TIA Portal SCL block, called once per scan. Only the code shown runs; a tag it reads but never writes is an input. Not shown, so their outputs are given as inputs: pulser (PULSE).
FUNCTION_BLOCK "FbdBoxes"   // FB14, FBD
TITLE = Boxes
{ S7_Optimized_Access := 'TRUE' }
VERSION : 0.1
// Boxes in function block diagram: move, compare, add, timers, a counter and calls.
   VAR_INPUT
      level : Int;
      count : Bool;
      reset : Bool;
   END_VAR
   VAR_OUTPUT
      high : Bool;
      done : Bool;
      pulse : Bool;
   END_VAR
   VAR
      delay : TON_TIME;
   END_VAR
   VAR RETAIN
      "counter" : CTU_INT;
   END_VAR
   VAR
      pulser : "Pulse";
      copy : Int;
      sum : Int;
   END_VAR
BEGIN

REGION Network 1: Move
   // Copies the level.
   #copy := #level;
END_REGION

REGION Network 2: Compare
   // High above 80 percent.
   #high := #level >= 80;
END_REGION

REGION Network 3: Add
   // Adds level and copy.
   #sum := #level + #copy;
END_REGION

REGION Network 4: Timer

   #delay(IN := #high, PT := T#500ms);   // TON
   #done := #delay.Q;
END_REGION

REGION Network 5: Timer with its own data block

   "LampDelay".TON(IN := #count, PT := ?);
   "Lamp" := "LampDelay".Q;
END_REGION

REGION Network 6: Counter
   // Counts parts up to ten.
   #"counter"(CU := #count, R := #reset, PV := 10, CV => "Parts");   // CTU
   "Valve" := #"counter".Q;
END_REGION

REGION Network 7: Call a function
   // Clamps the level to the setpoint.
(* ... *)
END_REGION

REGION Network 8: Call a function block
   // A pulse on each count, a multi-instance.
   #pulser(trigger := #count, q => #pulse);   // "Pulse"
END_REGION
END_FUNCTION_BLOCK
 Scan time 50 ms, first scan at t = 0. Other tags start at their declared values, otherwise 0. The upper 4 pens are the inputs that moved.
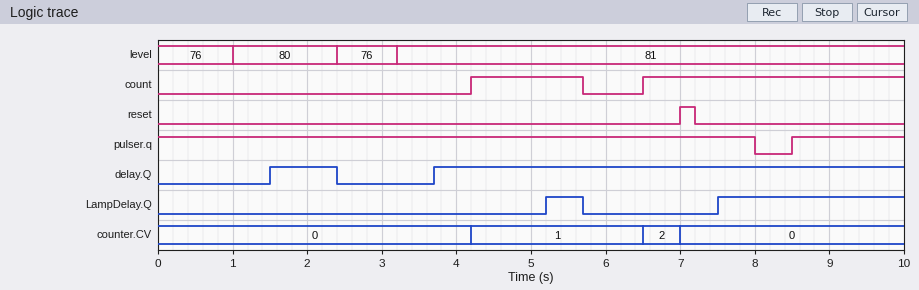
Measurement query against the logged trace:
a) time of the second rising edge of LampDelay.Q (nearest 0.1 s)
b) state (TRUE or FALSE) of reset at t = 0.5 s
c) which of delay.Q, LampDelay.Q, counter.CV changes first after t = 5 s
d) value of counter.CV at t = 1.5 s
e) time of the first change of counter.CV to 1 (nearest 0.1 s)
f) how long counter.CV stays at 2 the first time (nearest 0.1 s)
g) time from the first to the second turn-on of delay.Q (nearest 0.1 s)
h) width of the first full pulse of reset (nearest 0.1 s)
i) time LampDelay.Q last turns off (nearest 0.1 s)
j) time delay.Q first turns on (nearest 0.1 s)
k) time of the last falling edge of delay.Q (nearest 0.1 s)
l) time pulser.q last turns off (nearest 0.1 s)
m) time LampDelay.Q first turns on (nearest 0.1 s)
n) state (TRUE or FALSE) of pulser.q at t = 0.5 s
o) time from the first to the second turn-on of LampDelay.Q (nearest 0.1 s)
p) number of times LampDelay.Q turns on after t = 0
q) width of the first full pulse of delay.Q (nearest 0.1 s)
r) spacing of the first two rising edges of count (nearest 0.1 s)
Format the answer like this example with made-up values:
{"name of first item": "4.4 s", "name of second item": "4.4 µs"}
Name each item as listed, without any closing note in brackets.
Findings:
{"time of the second rising edge of LampDelay.Q": "7.5 s", "state (TRUE or FALSE) of reset at t = 0.5 s": "FALSE", "which of delay.Q, LampDelay.Q, counter.CV changes first after t = 5 s": "LampDelay.Q", "value of counter.CV at t = 1.5 s": "0", "time of the first change of counter.CV to 1": "4.2 s", "how long counter.CV stays at 2 the first time": "0.5 s", "time from the first to the second turn-on of delay.Q": "2.2 s", "width of the first full pulse of reset": "0.2 s", "time LampDelay.Q last turns off": "5.7 s", "time delay.Q first turns on": "1.5 s", "time of the last falling edge of delay.Q": "2.4 s", "time pulser.q last turns off": "8.0 s", "time LampDelay.Q first turns on": "5.2 s", "state (TRUE or FALSE) of pulser.q at t = 0.5 s": "TRUE", "time from the first to the second turn-on of LampDelay.Q": "2.3 s", "number of times LampDelay.Q turns on after t = 0": "2", "width of the first full pulse of delay.Q": "0.9 s", "spacing of the first two rising edges of count": "2.3 s"}
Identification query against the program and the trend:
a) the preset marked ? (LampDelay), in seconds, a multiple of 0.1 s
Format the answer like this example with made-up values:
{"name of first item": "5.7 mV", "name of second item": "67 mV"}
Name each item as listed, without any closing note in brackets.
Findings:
{"the preset marked ? (LampDelay), in seconds, a multiple of 0.1 s": "1.0 s"}
